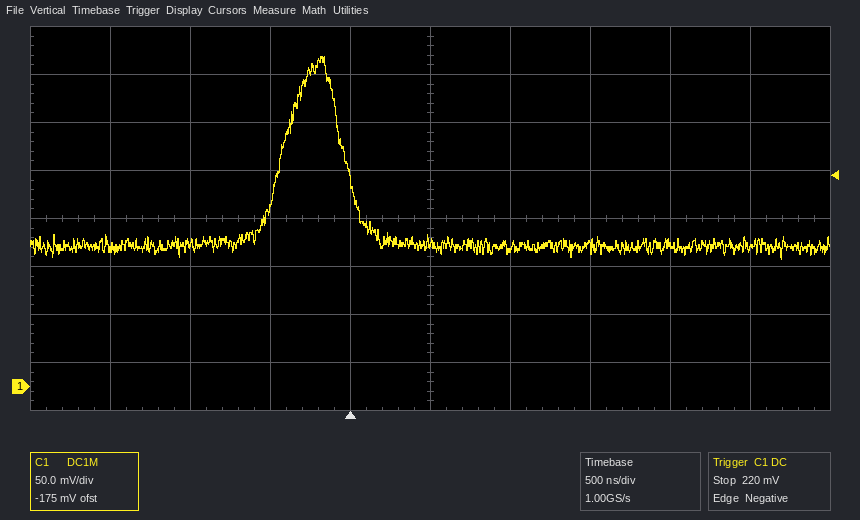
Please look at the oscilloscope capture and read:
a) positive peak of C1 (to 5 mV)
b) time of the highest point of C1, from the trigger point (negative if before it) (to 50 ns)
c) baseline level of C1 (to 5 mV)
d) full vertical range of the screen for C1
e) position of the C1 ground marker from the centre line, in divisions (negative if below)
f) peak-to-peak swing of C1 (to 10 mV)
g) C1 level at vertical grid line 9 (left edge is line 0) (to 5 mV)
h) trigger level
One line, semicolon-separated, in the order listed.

345 mV; -200 ns; 145 mV; 400 mV; -3.5 div; 210 mV; 145 mV; 220 mV
